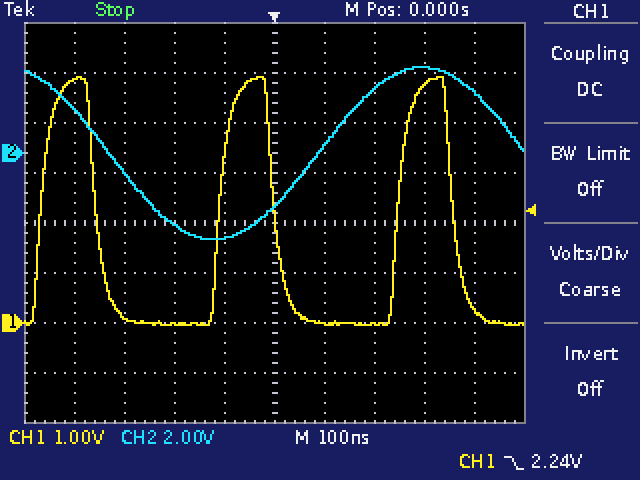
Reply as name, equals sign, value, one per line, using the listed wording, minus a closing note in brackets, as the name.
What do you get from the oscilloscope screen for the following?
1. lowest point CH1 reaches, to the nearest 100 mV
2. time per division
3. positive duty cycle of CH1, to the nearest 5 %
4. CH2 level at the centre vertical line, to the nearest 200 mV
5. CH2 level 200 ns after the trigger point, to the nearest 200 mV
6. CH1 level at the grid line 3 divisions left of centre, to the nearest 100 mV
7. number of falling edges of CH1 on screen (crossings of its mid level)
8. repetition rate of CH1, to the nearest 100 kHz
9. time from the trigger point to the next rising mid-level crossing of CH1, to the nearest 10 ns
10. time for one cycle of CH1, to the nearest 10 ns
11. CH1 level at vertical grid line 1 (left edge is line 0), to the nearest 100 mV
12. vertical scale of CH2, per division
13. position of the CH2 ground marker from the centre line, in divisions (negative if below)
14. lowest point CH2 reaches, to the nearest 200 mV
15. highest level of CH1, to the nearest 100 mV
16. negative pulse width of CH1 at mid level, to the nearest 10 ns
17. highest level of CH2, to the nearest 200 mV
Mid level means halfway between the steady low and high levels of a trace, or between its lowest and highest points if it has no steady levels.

lowest point CH1 reaches, to the nearest 100 mV = 0.0 V
time per division = 100 ns
positive duty cycle of CH1, to the nearest 5 % = 30 %
CH2 level at the centre vertical line, to the nearest 200 mV = -2.2 V
CH2 level 200 ns after the trigger point, to the nearest 200 mV = 2.6 V
CH1 level at the grid line 3 divisions left of centre, to the nearest 100 mV = 100 mV
number of falling edges of CH1 on screen = 3
repetition rate of CH1, to the nearest 100 kHz = 2.8 MHz
time from the trigger point to the next rising mid-level crossing of CH1, to the nearest 10 ns = 250 ns
time for one cycle of CH1, to the nearest 10 ns = 360 ns
CH1 level at vertical grid line 1 (left edge is line 0), to the nearest 100 mV = 4.9 V
vertical scale of CH2, per division = 2 V
position of the CH2 ground marker from the centre line, in divisions = +1.4 div
lowest point CH2 reaches, to the nearest 200 mV = -3.4 V
highest level of CH1, to the nearest 100 mV = 4.9 V
negative pulse width of CH1 at mid level, to the nearest 10 ns = 250 ns
highest level of CH2, to the nearest 200 mV = 3.4 V
